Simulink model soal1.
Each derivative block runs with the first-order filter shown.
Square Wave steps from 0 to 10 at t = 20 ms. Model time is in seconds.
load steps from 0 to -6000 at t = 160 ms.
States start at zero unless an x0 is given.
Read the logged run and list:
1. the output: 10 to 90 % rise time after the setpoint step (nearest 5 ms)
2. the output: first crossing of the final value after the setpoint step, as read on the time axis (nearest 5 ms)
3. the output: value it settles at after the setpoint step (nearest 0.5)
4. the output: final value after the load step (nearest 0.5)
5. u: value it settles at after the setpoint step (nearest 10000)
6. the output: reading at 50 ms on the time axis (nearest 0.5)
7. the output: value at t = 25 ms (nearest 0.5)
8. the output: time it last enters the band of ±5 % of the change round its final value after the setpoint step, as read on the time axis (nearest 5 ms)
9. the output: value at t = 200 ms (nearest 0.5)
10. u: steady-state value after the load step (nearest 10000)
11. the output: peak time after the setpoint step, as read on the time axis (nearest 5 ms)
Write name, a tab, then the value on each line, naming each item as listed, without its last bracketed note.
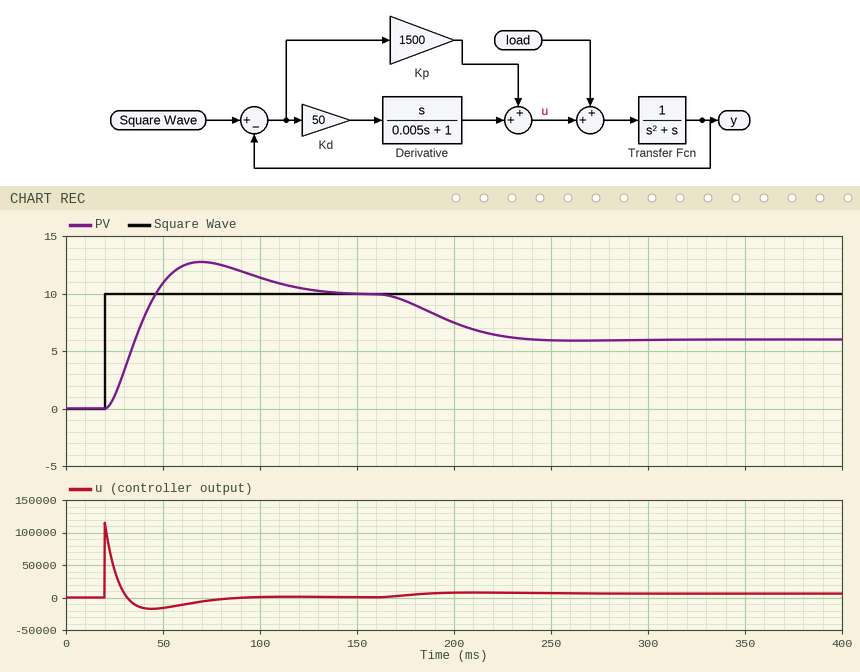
the output: 10 to 90 % rise time after the setpoint step	20 ms
the output: first crossing of the final value after the setpoint step, as read on the time axis	45 ms
the output: value it settles at after the setpoint step	10.0
the output: final value after the load step	6.0
u: value it settles at after the setpoint step	0
the output: reading at 50 ms on the time axis	11.0
the output: value at t = 25 ms	1.0
the output: time it last enters the band of ±5 % of the change round its final value after the setpoint step, as read on the time axis	120 ms
the output: value at t = 200 ms	7.5
u: steady-state value after the load step	10000
the output: peak time after the setpoint step, as read on the time axis	70 ms
